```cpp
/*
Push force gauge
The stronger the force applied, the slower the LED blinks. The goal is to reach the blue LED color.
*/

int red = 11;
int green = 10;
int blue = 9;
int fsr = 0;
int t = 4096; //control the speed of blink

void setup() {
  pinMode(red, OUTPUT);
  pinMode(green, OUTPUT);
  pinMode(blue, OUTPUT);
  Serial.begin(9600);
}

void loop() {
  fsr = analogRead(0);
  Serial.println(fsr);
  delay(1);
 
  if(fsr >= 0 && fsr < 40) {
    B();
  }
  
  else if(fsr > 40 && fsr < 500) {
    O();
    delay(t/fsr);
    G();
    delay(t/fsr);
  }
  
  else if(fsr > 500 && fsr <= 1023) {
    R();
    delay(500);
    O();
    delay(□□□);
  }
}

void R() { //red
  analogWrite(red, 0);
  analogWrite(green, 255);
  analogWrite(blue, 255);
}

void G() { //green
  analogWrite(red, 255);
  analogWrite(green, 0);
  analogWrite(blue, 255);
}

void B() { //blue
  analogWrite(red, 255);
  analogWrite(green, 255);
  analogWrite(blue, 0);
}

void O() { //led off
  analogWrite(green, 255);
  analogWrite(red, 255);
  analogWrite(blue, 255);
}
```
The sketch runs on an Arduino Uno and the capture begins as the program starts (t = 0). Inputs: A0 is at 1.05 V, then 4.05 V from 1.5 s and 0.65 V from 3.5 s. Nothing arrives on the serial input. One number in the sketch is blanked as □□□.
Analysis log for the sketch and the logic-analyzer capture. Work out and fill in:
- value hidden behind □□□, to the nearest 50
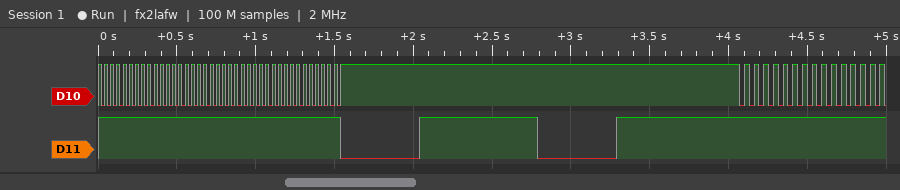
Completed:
750
